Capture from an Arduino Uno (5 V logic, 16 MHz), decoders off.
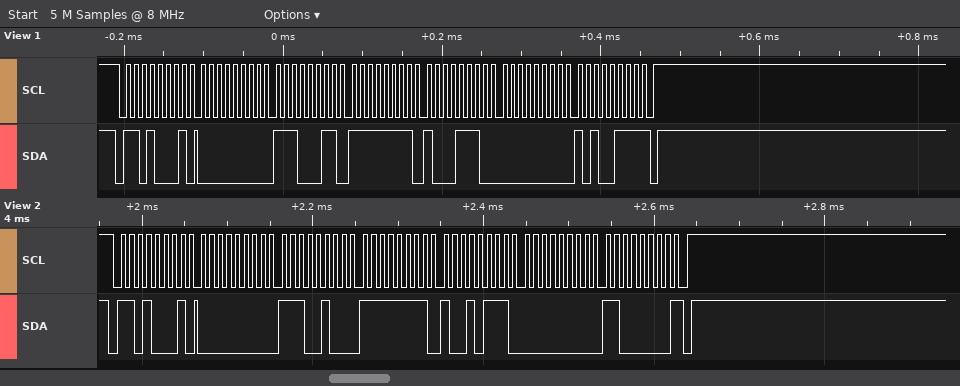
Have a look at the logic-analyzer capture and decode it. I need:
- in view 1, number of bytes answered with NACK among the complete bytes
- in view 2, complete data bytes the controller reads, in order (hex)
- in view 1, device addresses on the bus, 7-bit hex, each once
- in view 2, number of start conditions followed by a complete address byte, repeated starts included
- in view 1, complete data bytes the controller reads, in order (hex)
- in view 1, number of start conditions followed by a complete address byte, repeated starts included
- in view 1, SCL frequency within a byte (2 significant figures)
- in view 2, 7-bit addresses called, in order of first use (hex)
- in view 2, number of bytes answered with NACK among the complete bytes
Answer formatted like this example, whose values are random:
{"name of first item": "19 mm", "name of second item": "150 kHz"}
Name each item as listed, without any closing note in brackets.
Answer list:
{"in view 1, number of bytes answered with NACK among the complete bytes": "1", "in view 2, complete data bytes the controller reads, in order": "00 E4 FF 97 00 C0", "in view 1, device addresses on the bus, 7-bit hex, each once": "0x68", "in view 2, number of start conditions followed by a complete address byte, repeated starts included": "1", "in view 1, complete data bytes the controller reads, in order": "00 E3 FF 8E 00 A7", "in view 1, number of start conditions followed by a complete address byte, repeated starts included": "1", "in view 1, SCL frequency within a byte": "100 kHz", "in view 2, 7-bit addresses called, in order of first use": "0x68", "in view 2, number of bytes answered with NACK among the complete bytes": "1"}
